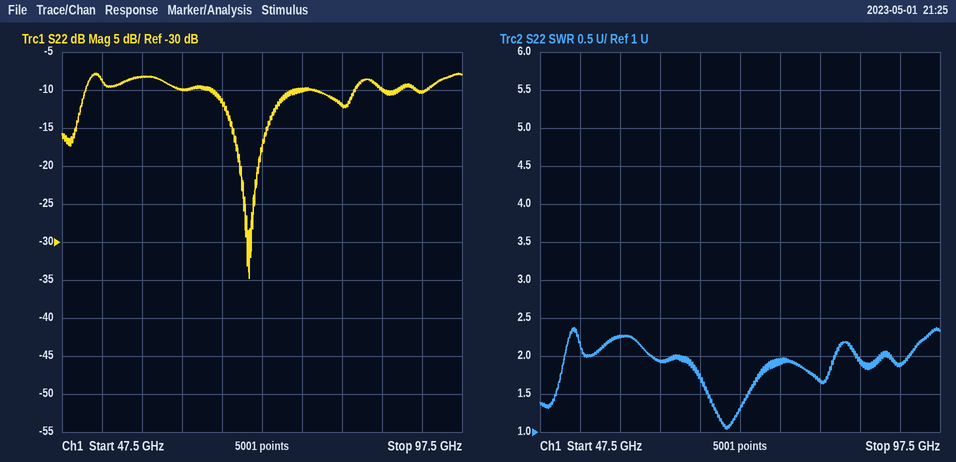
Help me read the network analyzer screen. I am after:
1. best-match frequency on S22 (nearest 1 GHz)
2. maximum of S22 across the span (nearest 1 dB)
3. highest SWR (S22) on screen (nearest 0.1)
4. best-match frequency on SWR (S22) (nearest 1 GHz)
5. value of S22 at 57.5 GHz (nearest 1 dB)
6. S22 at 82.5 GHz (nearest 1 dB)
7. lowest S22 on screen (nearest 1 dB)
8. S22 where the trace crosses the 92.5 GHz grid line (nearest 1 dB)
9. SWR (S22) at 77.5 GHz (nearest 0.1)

71 GHz
-8 dB
2.4
71 GHz
-8 dB
-12 dB
-35 dB
-10 dB
1.9
